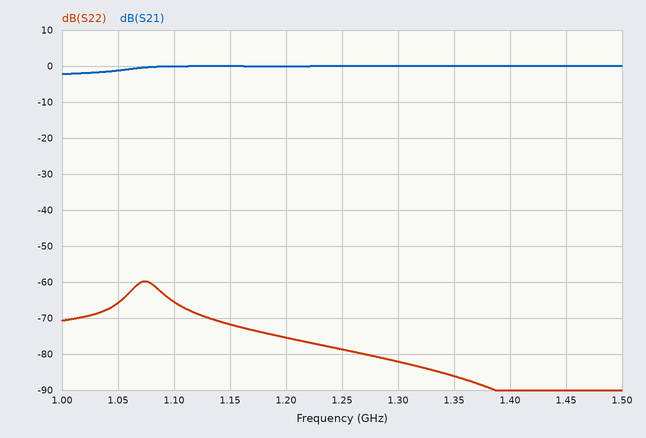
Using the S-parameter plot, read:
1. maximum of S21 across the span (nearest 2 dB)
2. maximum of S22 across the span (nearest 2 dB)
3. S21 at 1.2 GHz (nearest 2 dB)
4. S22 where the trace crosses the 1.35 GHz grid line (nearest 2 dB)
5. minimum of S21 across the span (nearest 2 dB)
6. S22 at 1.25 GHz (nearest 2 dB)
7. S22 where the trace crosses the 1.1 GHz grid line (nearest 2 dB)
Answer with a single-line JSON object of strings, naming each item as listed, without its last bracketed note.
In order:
{"maximum of S21 across the span": "0 dB", "maximum of S22 across the span": "-60 dB", "S21 at 1.2 GHz": "0 dB", "S22 where the trace crosses the 1.35 GHz grid line": "-86 dB", "minimum of S21 across the span": "-2 dB", "S22 at 1.25 GHz": "-78 dB", "S22 where the trace crosses the 1.1 GHz grid line": "-66 dB"}
